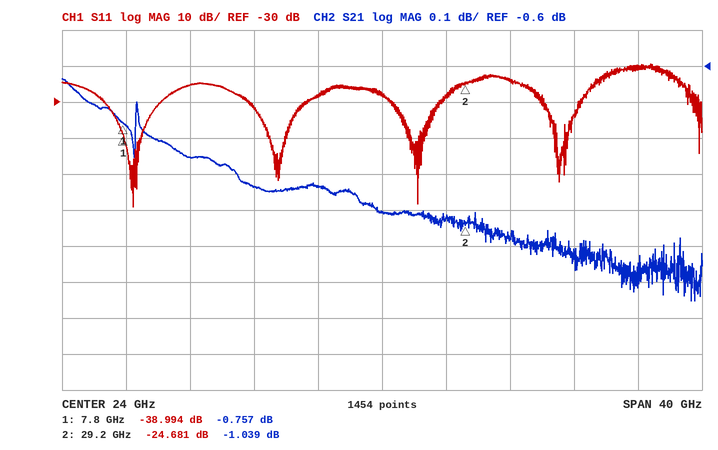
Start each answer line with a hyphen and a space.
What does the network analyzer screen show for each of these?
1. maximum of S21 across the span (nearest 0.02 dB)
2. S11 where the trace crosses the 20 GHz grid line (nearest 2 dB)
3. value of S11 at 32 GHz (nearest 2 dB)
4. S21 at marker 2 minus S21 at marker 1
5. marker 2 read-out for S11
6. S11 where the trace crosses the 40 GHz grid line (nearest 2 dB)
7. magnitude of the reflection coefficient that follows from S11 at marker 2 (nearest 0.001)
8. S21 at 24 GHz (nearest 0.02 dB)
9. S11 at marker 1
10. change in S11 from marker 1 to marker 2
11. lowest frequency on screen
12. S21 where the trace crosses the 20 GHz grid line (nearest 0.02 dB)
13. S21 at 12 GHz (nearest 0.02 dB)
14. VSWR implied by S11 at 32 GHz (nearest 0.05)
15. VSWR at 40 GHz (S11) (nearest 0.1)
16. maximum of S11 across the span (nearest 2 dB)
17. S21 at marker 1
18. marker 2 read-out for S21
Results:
- -0.64 dB
- -28 dB
- -24 dB
- -0.282 dB
- -24.681 dB
- -20 dB
- 0.058
- -1.00 dB
- -38.994 dB
- 14.313 dB
- 4 GHz
- -0.94 dB
- -0.86 dB
- 1.15
- 1.2
- -20 dB
- -0.757 dB
- -1.039 dB
